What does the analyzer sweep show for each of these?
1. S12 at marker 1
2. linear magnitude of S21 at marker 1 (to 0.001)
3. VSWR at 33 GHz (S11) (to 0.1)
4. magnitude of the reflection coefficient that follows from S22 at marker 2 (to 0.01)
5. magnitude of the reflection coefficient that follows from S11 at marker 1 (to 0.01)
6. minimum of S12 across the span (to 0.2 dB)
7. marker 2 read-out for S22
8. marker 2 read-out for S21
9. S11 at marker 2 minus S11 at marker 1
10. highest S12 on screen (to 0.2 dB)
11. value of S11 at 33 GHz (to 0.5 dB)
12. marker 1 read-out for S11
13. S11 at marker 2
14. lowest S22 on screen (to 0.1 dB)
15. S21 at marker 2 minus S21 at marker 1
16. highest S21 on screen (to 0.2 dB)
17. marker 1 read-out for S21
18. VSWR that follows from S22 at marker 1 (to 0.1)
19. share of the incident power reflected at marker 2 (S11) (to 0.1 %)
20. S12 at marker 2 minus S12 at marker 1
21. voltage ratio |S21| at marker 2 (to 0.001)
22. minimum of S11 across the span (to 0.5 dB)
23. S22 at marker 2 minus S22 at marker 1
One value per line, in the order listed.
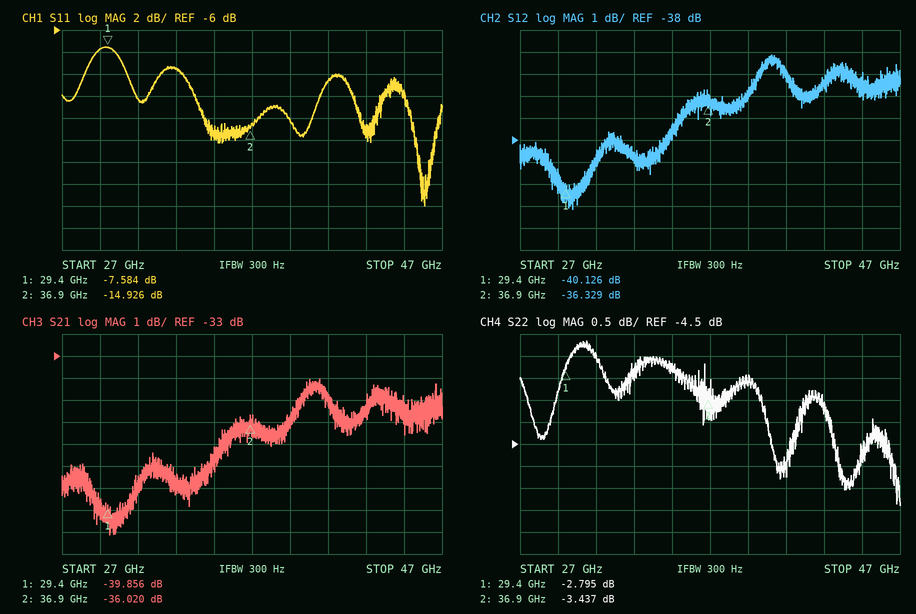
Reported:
-40.126 dB
0.010
2.0
0.67
0.42
-41.2 dB
-3.437 dB
-36.020 dB
-7.342 dB
-34.2 dB
-9.5 dB
-7.584 dB
-14.926 dB
-5.9 dB
3.836 dB
-34.0 dB
-39.856 dB
6.3
3.2 %
3.797 dB
0.016
-22.0 dB
-0.642 dB
